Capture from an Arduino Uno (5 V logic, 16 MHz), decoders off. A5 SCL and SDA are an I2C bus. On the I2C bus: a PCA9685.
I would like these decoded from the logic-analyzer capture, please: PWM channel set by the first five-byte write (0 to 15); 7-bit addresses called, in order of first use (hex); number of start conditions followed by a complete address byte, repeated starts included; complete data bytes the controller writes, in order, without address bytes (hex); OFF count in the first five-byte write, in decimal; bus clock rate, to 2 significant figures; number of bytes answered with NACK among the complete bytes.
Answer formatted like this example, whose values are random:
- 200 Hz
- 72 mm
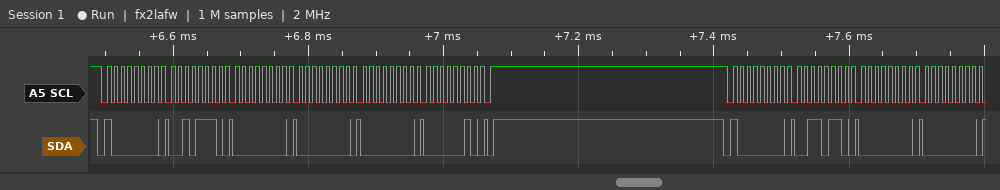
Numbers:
- 10
- 0x40
- 2
- 2E 00 00 00 02 36 00 00
- 512
- 100 kHz
- 0
